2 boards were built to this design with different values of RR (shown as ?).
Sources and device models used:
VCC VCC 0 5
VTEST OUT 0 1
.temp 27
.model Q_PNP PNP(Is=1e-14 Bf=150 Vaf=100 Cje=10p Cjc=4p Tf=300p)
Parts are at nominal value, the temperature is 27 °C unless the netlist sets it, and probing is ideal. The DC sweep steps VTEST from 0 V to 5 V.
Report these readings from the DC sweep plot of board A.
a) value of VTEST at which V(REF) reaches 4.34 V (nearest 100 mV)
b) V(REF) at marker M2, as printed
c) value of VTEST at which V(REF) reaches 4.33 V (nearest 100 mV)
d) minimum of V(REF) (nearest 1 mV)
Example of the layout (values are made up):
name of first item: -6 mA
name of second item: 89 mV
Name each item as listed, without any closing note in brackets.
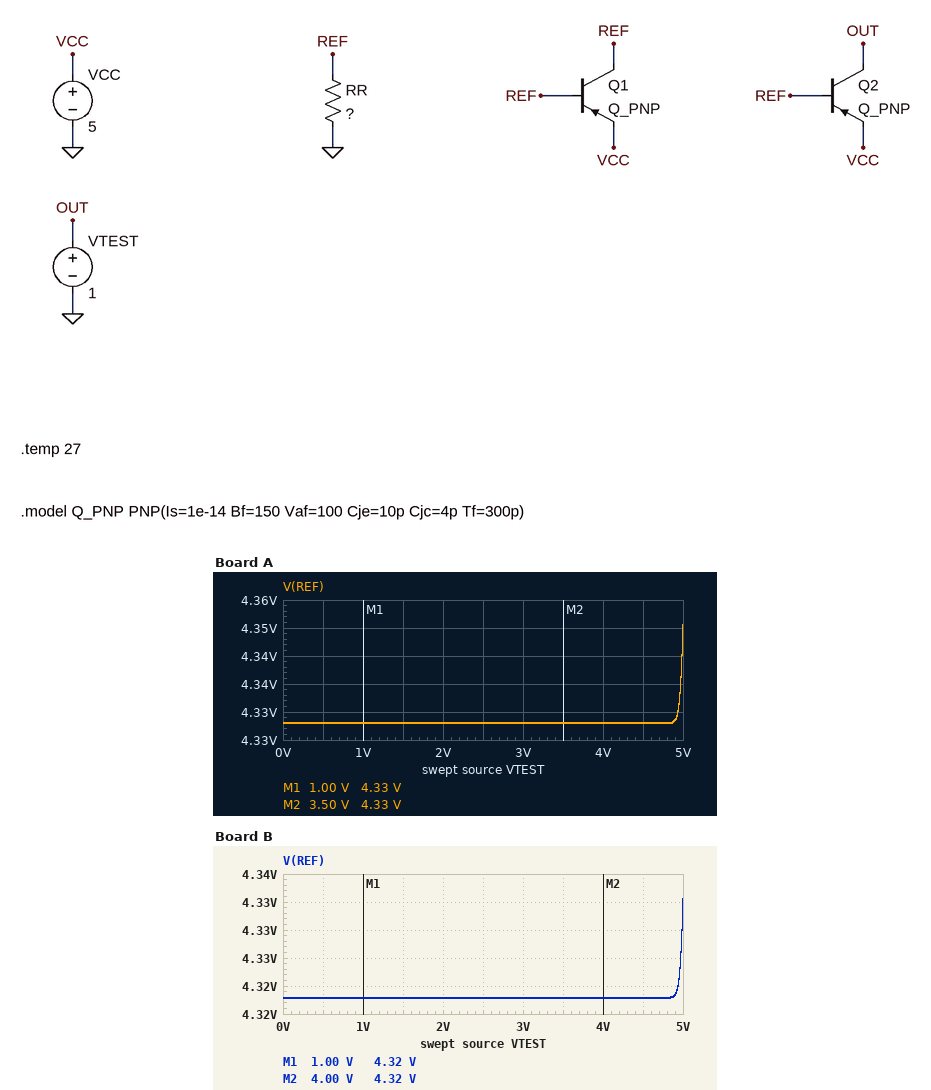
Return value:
value of VTEST at which V(REF) reaches 4.34 V: 5.0 V
V(REF) at marker M2, as printed: 4.33 V
value of VTEST at which V(REF) reaches 4.33 V: 4.9 V
minimum of V(REF): 4.333 V
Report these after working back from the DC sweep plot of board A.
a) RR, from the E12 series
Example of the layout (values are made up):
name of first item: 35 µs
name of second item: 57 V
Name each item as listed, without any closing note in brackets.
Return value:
RR, from the E12 series: 2.7 kΩ
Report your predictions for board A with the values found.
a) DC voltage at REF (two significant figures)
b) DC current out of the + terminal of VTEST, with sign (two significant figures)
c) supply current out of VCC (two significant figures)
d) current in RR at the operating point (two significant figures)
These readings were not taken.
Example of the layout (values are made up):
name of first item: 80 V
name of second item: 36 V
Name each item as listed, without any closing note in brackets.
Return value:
DC voltage at REF: 4.3 V
DC current out of the + terminal of VTEST, with sign: -1.6 mA
supply current out of VCC: 3.2 mA
current in RR at the operating point: 1.6 mA
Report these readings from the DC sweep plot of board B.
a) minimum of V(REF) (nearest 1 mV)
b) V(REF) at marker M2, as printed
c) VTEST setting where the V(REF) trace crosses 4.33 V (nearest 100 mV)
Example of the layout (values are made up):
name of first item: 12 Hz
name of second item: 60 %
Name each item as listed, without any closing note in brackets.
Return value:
minimum of V(REF): 4.318 V
V(REF) at marker M2, as printed: 4.32 V
VTEST setting where the V(REF) trace crosses 4.33 V: 5.0 V
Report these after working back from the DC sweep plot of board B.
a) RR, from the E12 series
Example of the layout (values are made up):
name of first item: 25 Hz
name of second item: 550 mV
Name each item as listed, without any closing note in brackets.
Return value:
RR, from the E12 series: 1.5 kΩ
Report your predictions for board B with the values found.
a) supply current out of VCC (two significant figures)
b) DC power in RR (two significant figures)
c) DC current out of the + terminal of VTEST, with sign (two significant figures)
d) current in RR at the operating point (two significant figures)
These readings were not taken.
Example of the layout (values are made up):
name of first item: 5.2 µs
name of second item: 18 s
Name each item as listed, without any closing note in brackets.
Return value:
supply current out of VCC: 5.8 mA
DC power in RR: 12 mW
DC current out of the + terminal of VTEST, with sign: -2.9 mA
current in RR at the operating point: 2.9 mA
